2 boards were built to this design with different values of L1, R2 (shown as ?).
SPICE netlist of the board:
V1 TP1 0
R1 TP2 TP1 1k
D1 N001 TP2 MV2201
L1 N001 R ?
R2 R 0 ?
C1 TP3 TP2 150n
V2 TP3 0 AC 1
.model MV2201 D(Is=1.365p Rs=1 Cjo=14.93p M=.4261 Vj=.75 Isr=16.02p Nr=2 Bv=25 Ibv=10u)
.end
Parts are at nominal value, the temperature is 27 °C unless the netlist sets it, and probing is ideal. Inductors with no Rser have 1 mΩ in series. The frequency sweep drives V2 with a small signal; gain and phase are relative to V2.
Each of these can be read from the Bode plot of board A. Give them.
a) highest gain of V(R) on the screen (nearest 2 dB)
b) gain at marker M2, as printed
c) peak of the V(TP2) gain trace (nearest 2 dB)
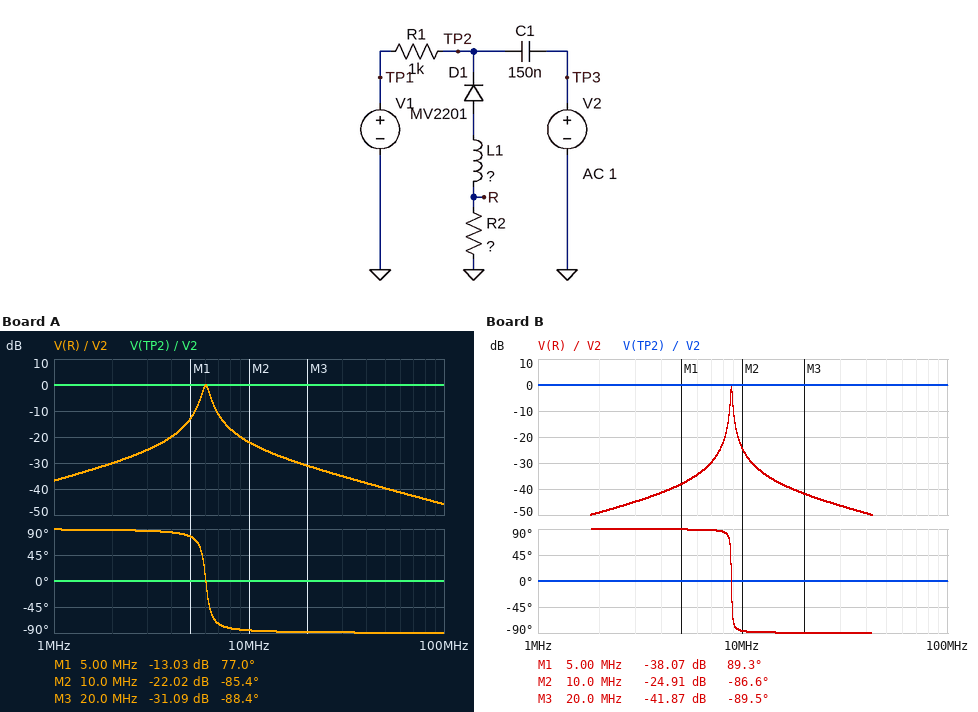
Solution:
0 dB
-22.02 dB
0 dB
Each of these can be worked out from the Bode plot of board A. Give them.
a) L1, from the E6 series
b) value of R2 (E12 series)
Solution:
47 µH
150 Ω
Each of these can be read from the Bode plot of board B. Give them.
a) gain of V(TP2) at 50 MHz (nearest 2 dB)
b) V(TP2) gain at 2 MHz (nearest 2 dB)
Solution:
0 dB
0 dB
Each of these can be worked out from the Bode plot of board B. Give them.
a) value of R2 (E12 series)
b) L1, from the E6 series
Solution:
18 Ω
22 µH
